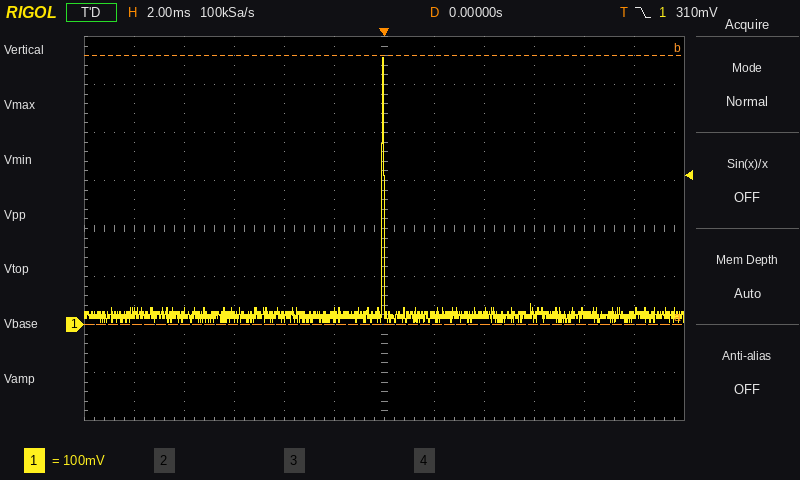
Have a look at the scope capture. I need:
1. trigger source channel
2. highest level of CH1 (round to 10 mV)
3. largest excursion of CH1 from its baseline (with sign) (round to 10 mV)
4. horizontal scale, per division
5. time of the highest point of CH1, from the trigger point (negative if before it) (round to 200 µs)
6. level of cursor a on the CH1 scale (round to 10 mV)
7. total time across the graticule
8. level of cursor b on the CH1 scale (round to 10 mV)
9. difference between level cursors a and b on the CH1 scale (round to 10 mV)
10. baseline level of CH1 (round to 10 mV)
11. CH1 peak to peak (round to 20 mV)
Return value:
CH1
560 mV
+540 mV
2 ms
0.0 ms
0 mV
24 ms
560 mV
560 mV
20 mV
560 mV
